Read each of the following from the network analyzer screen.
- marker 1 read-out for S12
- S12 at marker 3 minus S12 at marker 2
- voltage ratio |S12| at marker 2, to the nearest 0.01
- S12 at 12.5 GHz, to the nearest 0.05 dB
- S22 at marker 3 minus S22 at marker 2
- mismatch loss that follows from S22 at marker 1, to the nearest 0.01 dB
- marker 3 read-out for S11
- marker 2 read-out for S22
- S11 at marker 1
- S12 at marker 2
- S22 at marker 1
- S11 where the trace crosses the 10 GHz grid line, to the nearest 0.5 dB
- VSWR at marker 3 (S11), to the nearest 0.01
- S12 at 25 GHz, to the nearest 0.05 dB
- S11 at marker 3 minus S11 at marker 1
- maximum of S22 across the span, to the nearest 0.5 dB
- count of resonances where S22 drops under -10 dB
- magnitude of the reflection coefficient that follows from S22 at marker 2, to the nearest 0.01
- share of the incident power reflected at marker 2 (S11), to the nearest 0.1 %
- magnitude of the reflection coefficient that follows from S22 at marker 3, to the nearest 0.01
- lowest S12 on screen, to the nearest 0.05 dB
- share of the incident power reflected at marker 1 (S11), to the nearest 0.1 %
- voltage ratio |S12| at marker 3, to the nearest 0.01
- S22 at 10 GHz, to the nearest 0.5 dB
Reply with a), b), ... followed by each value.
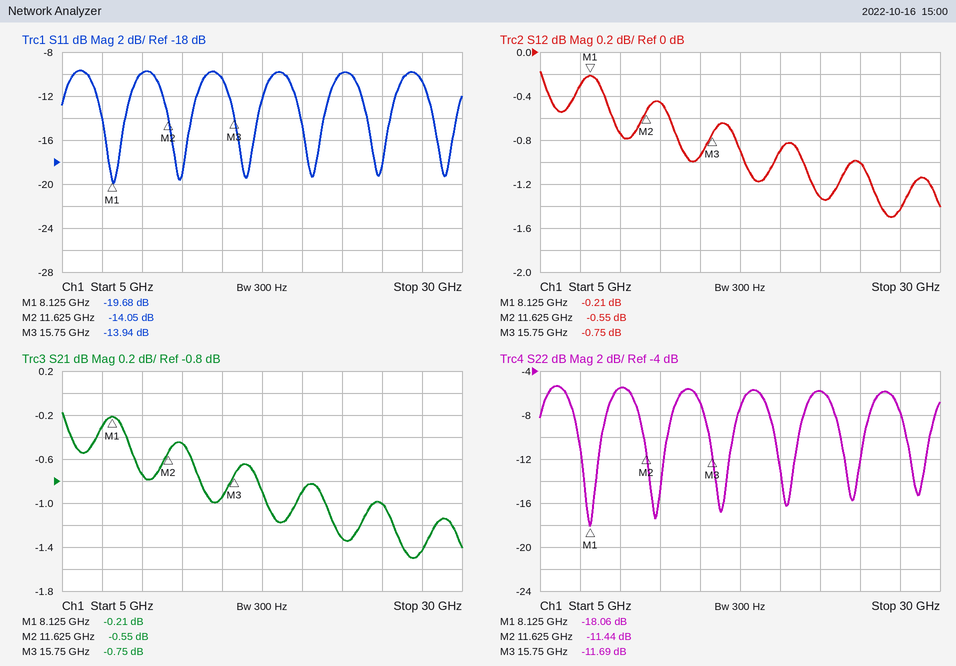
a) -0.21 dB
b) -0.20 dB
c) 0.94
d) -0.45 dB
e) -0.25 dB
f) 0.07 dB
g) -13.94 dB
h) -11.44 dB
i) -19.68 dB
j) -0.55 dB
k) -18.06 dB
l) -10.0 dB
m) 1.50
n) -1.00 dB
o) 5.74 dB
p) -5.5 dB
q) 6
r) 0.27
s) 3.9 %
t) 0.26
u) -1.50 dB
v) 1.1 %
w) 0.92
x) -5.5 dB
